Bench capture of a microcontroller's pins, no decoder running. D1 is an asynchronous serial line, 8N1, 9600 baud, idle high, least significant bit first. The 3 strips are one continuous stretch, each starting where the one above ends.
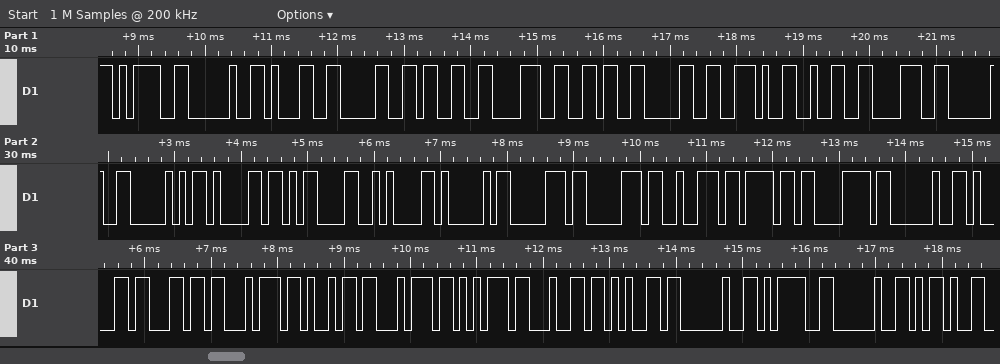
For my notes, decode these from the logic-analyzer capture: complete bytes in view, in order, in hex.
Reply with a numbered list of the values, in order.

1. 3D 20 31 30 33 38 36 30 2E 32 38 20 50 61 0D 0A 41 70 70 72 6F 78 20 61 6C 74 69 74 75 64 65 20 3D 20 2D
